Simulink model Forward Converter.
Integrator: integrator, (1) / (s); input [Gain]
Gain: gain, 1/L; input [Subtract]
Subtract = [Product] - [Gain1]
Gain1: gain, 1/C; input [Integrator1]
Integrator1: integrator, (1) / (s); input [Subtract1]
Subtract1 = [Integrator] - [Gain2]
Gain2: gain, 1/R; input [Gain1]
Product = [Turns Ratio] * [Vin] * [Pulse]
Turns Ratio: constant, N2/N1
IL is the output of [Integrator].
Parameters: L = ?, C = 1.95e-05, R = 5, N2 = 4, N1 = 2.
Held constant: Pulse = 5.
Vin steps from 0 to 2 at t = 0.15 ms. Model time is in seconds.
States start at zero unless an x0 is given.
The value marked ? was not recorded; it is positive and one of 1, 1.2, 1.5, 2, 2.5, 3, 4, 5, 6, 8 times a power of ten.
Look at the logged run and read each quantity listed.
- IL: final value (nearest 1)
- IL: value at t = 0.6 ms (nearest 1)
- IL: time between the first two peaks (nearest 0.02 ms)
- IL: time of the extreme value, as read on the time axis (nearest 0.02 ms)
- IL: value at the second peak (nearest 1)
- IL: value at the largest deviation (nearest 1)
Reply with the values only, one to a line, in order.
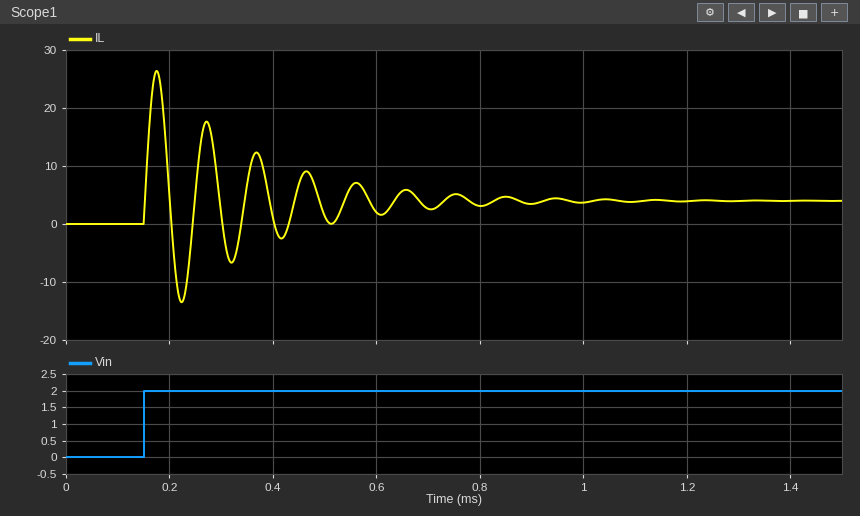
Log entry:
4
2
0.10 ms
0.18 ms
18
26
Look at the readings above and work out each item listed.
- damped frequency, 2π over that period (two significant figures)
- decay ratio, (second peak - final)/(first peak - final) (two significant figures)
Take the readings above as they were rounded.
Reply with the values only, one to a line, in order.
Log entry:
63 rad/ms
0.64
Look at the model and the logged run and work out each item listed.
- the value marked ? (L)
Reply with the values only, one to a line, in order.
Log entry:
1.2e-05
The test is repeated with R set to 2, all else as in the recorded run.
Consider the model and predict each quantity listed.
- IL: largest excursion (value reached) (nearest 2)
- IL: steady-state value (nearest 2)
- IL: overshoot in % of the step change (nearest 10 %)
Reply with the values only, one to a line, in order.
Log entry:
28
10
180 %
